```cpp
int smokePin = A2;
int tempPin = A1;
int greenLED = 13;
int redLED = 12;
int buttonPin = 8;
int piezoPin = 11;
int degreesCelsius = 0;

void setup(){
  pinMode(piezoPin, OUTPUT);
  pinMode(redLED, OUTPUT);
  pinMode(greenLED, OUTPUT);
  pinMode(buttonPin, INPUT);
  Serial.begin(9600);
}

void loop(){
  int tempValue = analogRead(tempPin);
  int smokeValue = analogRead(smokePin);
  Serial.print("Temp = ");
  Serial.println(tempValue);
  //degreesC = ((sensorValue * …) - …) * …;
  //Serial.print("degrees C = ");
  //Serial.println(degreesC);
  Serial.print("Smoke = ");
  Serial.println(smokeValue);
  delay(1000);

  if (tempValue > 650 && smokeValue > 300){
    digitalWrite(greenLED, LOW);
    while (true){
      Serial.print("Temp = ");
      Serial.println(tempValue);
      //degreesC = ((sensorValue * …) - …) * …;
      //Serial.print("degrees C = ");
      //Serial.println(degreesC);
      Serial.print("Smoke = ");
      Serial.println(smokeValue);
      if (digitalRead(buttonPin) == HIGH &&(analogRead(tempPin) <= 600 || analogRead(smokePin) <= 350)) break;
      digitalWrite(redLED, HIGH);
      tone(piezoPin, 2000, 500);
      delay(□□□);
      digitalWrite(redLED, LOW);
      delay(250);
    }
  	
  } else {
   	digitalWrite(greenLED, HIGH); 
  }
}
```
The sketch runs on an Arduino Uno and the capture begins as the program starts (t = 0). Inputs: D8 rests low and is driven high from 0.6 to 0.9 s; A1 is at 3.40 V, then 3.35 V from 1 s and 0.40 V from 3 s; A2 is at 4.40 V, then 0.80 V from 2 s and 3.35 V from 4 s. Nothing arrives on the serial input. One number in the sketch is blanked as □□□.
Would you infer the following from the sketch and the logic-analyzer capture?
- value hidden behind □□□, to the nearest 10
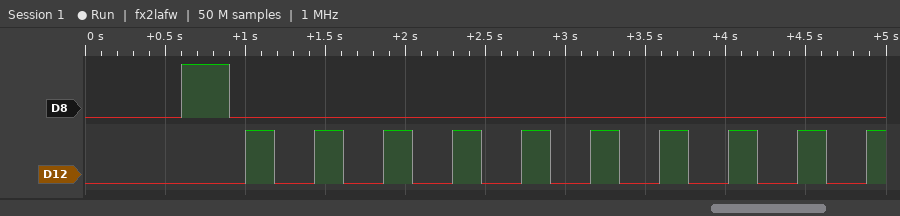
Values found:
180
